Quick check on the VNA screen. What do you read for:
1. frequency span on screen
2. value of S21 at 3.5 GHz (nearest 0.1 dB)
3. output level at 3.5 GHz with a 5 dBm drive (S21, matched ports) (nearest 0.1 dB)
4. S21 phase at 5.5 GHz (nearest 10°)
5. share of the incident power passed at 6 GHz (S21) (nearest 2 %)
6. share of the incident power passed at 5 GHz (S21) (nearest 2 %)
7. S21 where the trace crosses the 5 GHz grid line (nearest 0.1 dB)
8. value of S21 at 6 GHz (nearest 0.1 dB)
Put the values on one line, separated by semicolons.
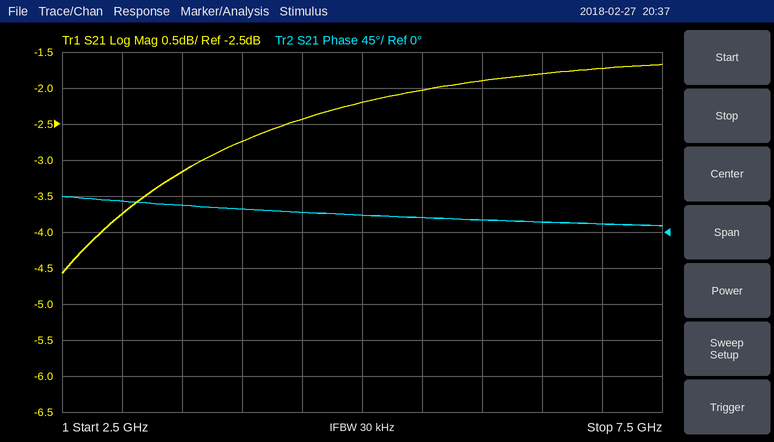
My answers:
5 GHz; -3.2 dB; 1.8 dBm; 20°; 64 %; 60 %; -2.2 dB; -1.9 dB
